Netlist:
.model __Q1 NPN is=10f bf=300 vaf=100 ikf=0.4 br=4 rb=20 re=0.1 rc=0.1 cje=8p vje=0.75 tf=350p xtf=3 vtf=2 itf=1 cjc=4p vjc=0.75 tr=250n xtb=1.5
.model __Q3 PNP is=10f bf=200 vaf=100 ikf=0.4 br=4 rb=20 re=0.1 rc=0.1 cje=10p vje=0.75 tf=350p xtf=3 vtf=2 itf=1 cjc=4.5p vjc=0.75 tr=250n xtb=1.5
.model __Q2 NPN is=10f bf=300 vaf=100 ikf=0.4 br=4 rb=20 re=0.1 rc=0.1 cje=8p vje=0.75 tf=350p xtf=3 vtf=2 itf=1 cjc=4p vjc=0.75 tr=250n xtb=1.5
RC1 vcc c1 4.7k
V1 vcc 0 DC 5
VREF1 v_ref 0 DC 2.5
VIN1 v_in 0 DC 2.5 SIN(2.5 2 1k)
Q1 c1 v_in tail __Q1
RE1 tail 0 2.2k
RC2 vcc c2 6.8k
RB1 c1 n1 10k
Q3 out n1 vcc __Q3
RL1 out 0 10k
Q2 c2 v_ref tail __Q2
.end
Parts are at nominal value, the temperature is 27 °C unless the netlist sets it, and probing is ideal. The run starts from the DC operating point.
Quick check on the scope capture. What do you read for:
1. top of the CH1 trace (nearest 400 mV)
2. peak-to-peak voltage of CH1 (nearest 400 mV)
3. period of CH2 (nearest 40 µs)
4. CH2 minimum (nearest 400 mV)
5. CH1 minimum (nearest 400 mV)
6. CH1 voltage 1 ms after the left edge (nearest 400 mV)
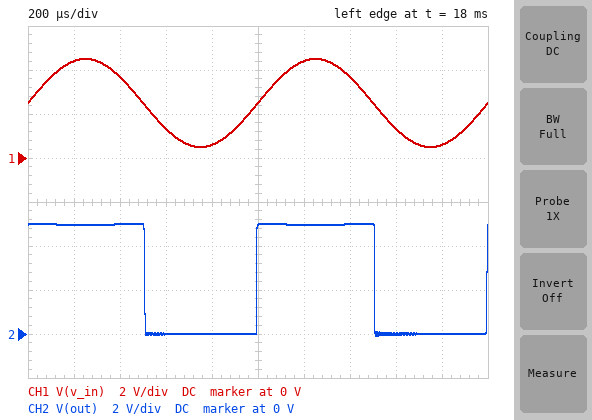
4.4 V
4.0 V
1.00 ms
0 V
400 mV
2.4 V
